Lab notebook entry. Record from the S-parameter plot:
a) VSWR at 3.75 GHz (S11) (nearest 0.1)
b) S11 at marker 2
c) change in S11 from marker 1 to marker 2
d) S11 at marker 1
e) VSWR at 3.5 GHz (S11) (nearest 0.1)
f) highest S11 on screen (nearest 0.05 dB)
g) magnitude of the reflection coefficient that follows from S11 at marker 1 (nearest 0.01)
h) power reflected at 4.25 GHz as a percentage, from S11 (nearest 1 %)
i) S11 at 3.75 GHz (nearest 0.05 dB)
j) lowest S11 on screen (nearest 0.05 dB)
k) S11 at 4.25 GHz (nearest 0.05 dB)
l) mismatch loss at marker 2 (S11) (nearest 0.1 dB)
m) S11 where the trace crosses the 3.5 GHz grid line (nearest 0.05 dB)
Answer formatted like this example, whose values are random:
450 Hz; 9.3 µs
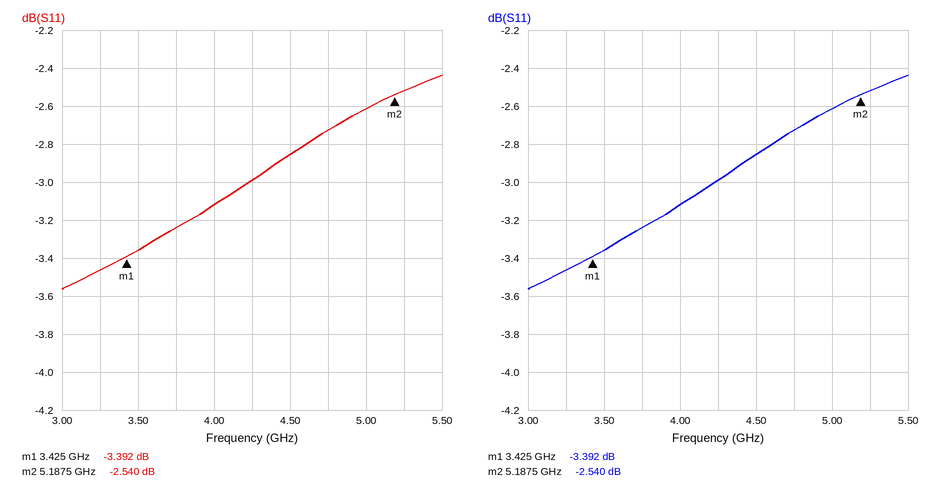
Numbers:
5.4; -2.540 dB; 0.852 dB; -3.392 dB; 5.2; -2.45 dB; 0.68; 50 %; -3.25 dB; -3.55 dB; -3.00 dB; 3.5 dB; -3.35 dB
